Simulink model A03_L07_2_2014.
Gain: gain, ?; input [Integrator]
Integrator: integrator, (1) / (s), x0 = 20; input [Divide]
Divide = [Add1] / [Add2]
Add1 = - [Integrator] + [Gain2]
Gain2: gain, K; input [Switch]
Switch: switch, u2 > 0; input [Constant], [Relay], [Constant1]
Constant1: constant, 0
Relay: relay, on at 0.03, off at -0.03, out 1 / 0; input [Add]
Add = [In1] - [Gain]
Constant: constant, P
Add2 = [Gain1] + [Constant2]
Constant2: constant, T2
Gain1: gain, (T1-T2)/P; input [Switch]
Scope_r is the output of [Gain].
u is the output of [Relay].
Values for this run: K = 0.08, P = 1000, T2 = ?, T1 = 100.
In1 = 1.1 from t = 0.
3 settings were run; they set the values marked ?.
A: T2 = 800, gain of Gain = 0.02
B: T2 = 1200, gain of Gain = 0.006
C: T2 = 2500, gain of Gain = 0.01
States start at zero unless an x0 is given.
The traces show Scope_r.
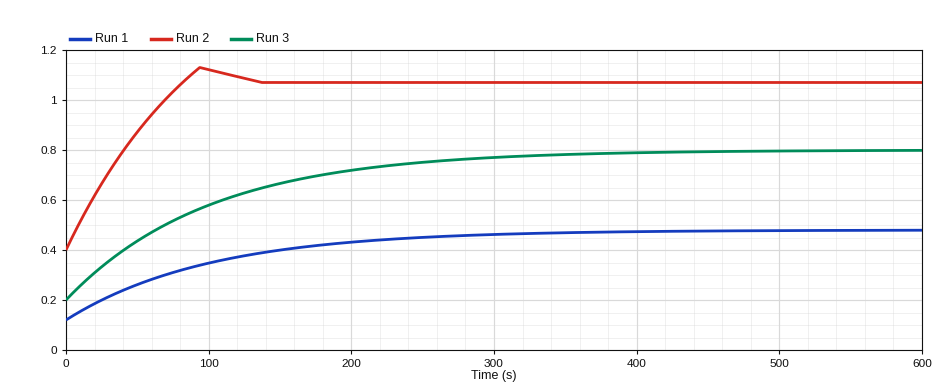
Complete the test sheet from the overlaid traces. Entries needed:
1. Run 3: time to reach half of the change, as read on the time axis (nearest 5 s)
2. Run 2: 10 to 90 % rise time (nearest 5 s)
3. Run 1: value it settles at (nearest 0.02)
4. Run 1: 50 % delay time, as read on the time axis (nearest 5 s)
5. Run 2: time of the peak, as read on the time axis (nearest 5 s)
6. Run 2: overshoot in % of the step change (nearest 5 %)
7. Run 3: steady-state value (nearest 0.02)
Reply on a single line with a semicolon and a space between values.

70 s; 65 s; 0.48; 70 s; 95 s; 10 %; 0.80
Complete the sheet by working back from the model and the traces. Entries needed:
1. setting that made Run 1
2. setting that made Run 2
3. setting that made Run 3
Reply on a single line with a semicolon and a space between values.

B; A; C
